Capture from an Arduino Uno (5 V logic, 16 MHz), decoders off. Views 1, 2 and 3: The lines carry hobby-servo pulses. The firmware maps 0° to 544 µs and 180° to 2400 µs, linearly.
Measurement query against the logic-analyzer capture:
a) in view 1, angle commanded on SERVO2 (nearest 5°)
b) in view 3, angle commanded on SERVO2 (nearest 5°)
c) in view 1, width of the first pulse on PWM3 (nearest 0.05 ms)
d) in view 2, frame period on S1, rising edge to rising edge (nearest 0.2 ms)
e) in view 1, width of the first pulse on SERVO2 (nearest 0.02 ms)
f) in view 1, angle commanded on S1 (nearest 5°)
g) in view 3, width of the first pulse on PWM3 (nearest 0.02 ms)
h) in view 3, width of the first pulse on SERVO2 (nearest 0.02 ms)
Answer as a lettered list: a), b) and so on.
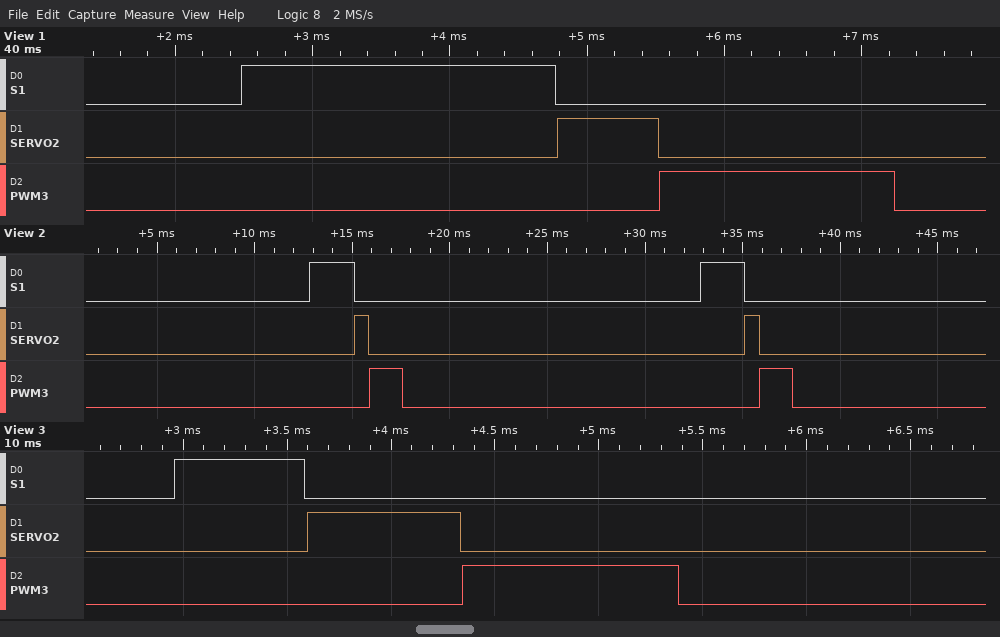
a) 20°
b) 20°
c) 1.70 ms
d) 20.0 ms
e) 0.74 ms
f) 170°
g) 1.04 ms
h) 0.74 ms
